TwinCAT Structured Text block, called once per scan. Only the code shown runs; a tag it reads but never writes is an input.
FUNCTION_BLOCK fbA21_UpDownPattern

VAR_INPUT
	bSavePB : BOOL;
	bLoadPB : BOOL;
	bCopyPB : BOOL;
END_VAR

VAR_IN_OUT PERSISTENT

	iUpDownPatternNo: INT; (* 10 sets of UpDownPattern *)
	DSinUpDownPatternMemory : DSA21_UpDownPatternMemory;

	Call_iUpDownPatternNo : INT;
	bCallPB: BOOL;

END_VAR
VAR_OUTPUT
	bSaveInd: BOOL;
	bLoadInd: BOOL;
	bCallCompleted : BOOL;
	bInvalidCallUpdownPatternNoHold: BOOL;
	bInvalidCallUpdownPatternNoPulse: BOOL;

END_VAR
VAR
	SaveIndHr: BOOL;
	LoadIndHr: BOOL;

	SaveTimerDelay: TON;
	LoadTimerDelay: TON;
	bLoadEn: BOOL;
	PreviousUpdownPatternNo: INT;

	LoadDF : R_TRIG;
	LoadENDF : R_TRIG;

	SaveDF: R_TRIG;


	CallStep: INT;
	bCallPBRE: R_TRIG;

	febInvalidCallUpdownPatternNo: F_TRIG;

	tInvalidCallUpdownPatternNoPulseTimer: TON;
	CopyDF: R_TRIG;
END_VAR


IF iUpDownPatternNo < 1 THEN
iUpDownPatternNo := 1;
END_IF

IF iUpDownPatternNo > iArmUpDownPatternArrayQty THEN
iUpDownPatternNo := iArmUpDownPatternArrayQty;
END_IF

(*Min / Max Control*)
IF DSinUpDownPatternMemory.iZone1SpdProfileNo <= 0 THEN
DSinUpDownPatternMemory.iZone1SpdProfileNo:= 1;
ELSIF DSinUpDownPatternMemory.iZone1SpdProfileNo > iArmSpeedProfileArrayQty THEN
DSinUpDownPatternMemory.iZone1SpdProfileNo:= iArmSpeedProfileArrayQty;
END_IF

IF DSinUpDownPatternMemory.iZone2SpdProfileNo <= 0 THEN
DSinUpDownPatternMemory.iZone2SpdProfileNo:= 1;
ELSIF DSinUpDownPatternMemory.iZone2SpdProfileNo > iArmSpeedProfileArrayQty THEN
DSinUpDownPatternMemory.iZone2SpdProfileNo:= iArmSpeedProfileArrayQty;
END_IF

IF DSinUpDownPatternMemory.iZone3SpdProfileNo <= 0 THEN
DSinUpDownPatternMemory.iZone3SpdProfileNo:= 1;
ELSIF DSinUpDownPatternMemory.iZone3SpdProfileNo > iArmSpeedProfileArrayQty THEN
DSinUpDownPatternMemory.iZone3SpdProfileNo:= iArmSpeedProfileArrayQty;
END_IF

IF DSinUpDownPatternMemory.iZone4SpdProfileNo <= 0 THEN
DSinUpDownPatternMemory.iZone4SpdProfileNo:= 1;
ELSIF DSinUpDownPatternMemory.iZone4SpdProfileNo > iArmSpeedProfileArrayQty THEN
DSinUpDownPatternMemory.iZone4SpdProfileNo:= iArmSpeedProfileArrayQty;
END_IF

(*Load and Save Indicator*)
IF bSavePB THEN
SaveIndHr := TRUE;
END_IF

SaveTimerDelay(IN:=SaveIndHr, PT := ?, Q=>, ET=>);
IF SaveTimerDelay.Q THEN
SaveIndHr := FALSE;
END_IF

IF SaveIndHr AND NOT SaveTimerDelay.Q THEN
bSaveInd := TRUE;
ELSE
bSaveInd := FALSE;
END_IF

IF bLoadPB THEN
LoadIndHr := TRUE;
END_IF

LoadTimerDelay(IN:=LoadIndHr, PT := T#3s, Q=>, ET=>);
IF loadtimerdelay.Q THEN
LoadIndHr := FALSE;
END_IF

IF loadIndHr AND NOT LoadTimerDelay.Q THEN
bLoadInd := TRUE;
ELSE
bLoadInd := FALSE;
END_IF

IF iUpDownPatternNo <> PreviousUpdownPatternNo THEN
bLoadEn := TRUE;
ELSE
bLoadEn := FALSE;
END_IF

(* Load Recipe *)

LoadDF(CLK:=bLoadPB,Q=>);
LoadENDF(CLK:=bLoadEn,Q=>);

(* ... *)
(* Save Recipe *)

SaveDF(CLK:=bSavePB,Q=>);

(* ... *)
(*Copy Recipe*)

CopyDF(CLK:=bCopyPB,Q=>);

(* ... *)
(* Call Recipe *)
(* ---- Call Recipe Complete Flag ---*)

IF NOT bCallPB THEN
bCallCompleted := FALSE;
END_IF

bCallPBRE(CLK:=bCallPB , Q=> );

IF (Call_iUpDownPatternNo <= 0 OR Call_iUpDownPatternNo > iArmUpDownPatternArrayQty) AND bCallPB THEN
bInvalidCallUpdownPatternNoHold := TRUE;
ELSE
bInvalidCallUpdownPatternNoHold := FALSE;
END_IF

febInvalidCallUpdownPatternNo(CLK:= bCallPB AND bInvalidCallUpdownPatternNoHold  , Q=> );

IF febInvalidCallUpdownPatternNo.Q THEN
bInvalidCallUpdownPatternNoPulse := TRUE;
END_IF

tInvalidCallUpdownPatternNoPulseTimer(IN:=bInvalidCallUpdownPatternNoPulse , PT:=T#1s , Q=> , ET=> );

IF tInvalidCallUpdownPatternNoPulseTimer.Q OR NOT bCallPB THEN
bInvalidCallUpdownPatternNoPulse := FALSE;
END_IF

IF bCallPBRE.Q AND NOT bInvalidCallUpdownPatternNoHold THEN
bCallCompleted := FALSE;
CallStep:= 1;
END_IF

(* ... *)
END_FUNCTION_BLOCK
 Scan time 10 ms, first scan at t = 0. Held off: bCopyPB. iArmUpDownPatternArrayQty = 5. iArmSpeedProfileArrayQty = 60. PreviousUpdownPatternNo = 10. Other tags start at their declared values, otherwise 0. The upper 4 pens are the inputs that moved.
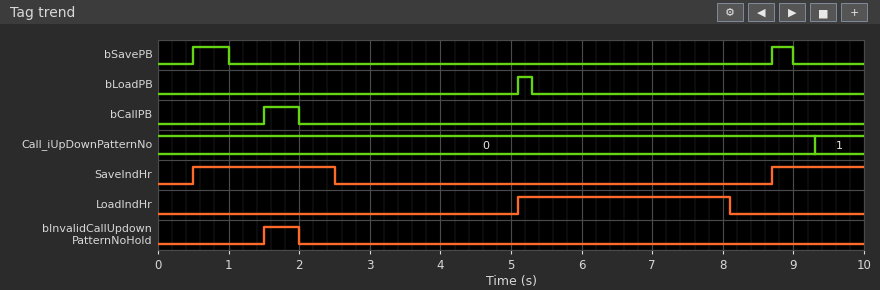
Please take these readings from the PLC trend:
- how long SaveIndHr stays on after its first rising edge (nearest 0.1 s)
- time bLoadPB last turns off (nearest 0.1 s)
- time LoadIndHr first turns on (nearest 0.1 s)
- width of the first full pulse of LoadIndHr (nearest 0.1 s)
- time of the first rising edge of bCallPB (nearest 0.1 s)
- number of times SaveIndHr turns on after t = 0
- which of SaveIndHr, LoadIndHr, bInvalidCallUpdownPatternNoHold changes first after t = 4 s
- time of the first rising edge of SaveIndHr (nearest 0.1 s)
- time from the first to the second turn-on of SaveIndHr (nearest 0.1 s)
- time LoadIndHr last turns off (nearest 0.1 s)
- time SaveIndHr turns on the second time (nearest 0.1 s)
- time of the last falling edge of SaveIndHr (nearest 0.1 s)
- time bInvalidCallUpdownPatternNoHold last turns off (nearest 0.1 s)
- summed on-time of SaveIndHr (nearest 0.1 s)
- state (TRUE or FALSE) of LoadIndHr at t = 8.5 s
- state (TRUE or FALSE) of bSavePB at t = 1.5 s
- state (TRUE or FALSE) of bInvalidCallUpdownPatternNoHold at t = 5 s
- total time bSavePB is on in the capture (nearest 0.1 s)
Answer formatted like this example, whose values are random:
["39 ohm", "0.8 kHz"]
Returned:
["2.0 s", "5.3 s", "5.1 s", "3.0 s", "1.5 s", "2", "LoadIndHr", "0.5 s", "8.2 s", "8.1 s", "8.7 s", "2.5 s", "2.0 s", "3.3 s", "FALSE", "FALSE", "FALSE", "0.8 s"]
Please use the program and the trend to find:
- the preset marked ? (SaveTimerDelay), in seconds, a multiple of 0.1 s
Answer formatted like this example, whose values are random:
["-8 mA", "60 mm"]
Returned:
["2.0 s"]
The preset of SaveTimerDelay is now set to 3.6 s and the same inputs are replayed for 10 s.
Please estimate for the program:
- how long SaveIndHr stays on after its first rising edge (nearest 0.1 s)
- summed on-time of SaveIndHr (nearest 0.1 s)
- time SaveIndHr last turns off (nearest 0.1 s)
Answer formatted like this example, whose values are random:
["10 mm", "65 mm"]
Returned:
["3.6 s", "4.9 s", "4.1 s"]
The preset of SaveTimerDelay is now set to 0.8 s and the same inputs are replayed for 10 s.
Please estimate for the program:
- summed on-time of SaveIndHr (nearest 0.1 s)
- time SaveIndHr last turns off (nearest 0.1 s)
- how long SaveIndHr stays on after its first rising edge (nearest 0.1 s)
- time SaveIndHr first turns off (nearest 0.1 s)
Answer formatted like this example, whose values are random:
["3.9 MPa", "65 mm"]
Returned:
["1.6 s", "9.5 s", "0.8 s", "1.3 s"]
